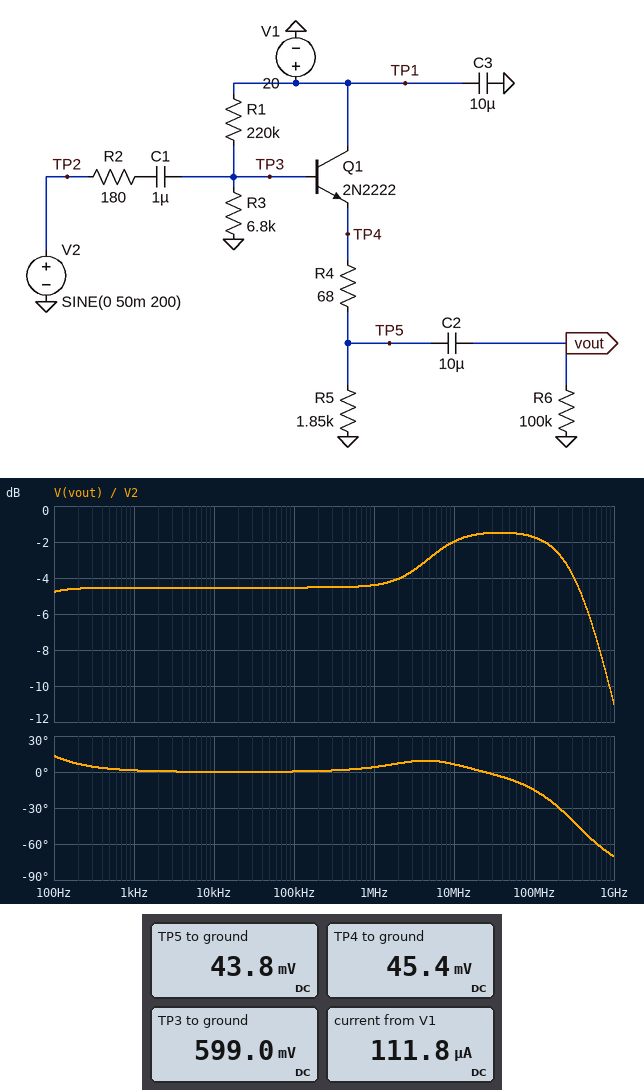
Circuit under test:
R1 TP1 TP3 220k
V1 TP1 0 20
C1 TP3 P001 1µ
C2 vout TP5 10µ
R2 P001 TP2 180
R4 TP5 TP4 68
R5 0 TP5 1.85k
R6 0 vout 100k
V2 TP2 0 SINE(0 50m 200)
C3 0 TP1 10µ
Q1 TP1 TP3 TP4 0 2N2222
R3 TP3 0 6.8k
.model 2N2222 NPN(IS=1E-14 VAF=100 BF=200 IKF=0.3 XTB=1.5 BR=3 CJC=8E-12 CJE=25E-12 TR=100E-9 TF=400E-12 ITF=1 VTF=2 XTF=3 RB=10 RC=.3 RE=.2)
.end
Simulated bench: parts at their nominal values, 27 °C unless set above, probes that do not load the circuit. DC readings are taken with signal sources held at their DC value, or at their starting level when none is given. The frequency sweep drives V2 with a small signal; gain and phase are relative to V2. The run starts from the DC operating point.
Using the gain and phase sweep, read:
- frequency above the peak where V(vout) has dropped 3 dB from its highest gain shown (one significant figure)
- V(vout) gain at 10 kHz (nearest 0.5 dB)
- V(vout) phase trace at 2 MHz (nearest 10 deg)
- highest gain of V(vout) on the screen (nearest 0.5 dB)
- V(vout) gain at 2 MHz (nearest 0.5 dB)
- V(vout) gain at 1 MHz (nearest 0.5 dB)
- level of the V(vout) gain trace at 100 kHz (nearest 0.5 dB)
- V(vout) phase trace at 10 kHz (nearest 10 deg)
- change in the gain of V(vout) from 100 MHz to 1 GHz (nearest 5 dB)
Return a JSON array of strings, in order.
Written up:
["400 MHz", "-4.5 dB", "10 deg", "-1.5 dB", "-4.0 dB", "-4.5 dB", "-4.5 dB", "0 deg", "-10 dB"]
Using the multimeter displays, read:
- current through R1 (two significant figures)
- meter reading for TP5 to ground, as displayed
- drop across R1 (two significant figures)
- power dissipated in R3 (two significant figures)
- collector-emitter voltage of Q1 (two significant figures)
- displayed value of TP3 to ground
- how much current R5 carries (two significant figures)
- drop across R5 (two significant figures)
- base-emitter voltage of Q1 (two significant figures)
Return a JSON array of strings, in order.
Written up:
["88 µA", "43.8 mV", "19 V", "53 µW", "20 V", "599.0 mV", "24 µA", "44 mV", "550 mV"]
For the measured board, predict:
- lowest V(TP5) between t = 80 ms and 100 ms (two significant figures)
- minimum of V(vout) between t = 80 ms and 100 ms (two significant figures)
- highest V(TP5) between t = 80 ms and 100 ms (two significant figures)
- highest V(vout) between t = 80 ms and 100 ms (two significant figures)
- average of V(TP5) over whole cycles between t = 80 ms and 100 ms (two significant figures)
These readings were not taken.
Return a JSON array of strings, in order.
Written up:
["19 mV", "-25 mV", "76 mV", "32 mV", "46 mV"]
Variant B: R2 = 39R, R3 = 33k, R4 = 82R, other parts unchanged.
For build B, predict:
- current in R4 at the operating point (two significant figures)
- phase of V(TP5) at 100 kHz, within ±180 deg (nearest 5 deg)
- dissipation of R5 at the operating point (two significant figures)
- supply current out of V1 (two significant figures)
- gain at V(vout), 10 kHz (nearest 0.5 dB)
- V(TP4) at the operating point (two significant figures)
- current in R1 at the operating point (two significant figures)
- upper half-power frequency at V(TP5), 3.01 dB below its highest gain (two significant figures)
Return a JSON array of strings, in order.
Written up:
["950 µA", "0 deg", "1.7 mW", "1.0 mA", "-0.5 dB", "1.8 V", "80 µA", "1.2 GHz"]
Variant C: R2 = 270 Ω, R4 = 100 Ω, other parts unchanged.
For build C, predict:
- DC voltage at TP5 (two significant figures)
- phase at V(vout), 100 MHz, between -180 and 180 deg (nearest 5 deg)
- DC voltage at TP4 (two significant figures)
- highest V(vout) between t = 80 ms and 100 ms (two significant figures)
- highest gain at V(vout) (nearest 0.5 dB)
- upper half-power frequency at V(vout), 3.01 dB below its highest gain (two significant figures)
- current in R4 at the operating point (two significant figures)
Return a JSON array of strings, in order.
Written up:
["43 mV", "-20 deg", "46 mV", "31 mV", "-2.0 dB", "260 MHz", "23 µA"]
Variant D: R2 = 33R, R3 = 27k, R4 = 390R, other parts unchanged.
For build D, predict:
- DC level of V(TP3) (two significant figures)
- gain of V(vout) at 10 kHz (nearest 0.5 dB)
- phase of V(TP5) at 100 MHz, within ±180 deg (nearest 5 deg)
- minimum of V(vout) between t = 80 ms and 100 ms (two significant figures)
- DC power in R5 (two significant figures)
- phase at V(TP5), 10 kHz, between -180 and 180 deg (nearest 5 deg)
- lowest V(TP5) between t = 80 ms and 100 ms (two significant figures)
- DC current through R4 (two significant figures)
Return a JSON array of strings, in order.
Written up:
["2.1 V", "-2.0 dB", "-5 deg", "-40 mV", "810 µW", "0 deg", "1.2 V", "660 µA"]
